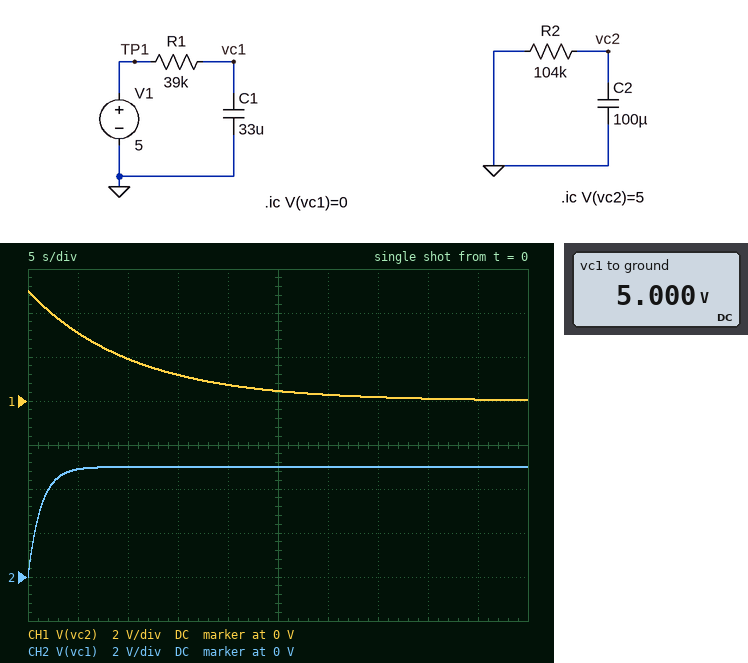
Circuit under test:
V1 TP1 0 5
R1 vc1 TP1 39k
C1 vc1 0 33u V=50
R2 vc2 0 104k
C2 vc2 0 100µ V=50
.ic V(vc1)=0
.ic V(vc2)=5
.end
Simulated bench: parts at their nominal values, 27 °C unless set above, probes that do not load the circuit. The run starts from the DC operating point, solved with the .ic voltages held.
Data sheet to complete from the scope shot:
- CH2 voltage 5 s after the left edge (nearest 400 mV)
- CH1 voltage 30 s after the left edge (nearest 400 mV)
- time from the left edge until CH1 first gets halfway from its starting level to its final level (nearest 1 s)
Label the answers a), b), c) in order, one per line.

a) 4.8 V
b) 400 mV
c) 7 s
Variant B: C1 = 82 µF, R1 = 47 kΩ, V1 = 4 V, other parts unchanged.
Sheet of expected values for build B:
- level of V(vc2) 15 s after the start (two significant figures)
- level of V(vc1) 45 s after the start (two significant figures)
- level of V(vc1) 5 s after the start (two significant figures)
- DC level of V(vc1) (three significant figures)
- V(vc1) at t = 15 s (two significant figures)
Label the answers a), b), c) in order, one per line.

a) 1.2 V
b) 4.0 V
c) 2.9 V
d) 4.00 V
e) 3.9 V
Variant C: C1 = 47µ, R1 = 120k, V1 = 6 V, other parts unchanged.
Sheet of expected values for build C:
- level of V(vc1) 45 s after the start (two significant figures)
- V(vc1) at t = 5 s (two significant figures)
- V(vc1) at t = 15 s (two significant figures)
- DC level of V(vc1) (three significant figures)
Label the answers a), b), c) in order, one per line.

a) 6.0 V
b) 3.5 V
c) 5.6 V
d) 6.00 V
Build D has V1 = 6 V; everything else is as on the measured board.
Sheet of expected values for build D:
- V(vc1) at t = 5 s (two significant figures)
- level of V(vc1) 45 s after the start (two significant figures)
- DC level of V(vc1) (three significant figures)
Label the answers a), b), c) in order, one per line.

a) 5.9 V
b) 6.0 V
c) 6.00 V
